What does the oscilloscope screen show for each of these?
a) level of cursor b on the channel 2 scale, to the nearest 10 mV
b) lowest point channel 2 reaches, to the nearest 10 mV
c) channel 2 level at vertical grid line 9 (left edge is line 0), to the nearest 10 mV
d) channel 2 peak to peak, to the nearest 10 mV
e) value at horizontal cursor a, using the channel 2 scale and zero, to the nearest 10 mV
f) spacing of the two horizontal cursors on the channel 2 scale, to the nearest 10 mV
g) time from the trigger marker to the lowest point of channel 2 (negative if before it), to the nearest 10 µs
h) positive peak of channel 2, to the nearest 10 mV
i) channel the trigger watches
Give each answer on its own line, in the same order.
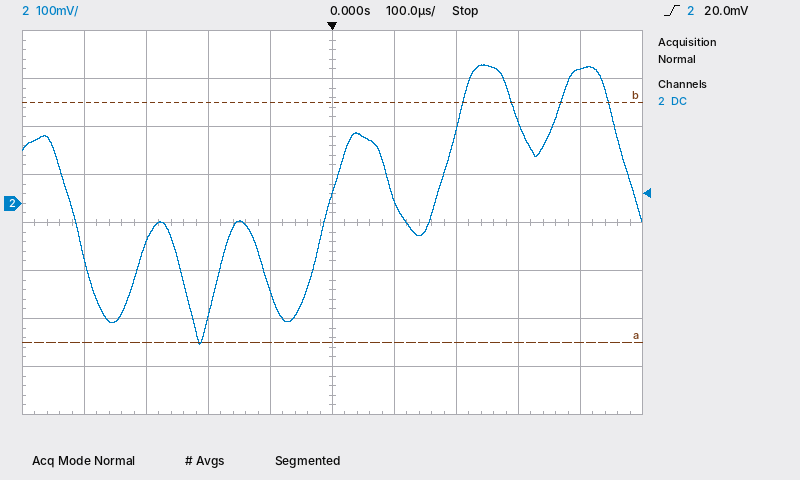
210 mV
-290 mV
280 mV
580 mV
-290 mV
500 mV
-210 µs
290 mV
channel 2
